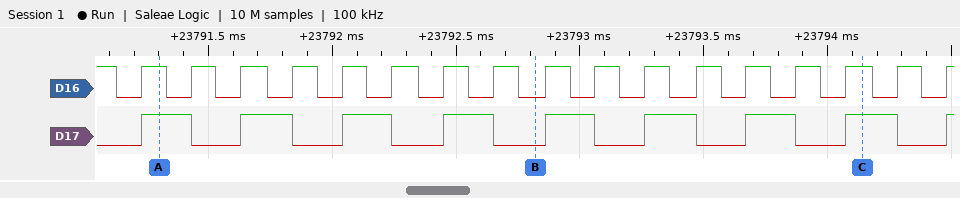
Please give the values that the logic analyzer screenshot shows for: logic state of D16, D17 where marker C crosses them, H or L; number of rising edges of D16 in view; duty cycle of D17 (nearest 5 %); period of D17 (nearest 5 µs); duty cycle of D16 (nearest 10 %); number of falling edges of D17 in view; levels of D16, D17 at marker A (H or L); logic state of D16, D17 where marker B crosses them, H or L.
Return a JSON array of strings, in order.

["D16=H, D17=H", "17", "50 %", "405 µs", "50 %", "8", "D16=H, D17=H", "D16=L, D17=L"]
